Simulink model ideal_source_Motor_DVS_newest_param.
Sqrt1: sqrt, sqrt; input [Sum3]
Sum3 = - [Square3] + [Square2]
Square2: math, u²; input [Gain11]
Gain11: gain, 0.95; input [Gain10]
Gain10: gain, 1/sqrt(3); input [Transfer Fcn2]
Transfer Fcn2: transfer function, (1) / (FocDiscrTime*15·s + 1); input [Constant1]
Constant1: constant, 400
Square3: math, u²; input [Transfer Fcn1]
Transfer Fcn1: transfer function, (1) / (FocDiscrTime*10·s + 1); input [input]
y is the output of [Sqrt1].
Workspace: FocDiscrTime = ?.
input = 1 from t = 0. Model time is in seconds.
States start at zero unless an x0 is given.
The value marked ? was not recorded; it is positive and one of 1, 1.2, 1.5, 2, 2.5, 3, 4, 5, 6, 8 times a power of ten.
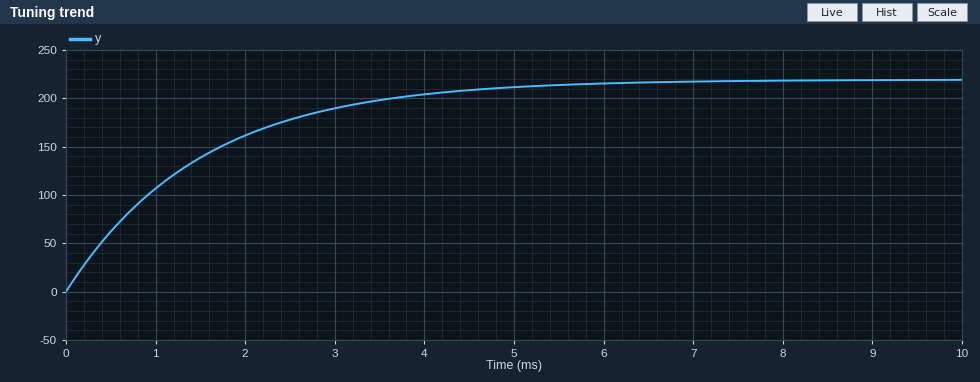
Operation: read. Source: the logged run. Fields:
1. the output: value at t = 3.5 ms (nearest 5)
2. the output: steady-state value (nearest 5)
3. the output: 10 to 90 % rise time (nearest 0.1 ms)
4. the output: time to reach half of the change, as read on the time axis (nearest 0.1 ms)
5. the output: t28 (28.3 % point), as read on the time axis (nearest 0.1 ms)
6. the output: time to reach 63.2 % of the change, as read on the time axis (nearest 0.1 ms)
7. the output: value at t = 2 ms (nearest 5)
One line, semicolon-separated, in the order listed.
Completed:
200; 220; 3.3 ms; 1.0 ms; 0.5 ms; 1.5 ms; 160
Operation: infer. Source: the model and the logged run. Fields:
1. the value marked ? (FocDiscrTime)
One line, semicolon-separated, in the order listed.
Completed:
0.0001
